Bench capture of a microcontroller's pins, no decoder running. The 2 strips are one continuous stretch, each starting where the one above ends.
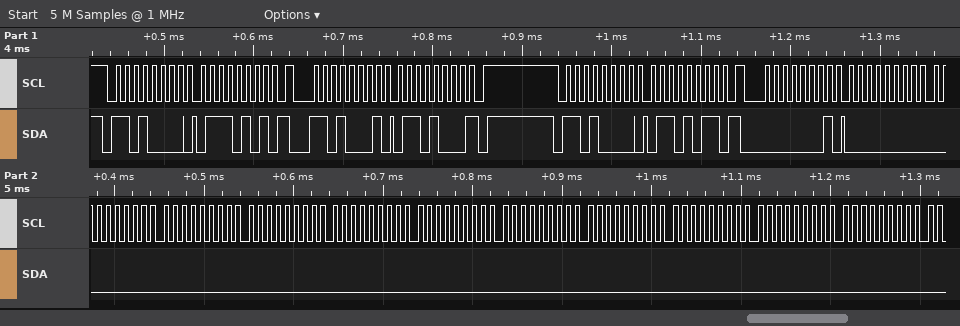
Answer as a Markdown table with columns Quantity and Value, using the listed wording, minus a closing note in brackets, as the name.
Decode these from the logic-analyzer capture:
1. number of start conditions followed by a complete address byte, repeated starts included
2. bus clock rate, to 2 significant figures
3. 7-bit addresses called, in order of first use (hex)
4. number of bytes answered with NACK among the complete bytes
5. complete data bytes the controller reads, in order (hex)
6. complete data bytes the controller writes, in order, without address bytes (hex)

| Quantity | Value |
|---|---|
| number of start conditions followed by a complete address byte, repeated starts included | 4 |
| bus clock rate, to 2 significant figures | 100 kHz |
| 7-bit addresses called, in order of first use | 0x68 0x00 |
| number of bytes answered with NACK among the complete bytes | 1 |
| complete data bytes the controller reads, in order | 68 00 00 00 00 00 00 00 00 00 00 00 |
| complete data bytes the controller writes, in order, without address bytes | 75 6B |
